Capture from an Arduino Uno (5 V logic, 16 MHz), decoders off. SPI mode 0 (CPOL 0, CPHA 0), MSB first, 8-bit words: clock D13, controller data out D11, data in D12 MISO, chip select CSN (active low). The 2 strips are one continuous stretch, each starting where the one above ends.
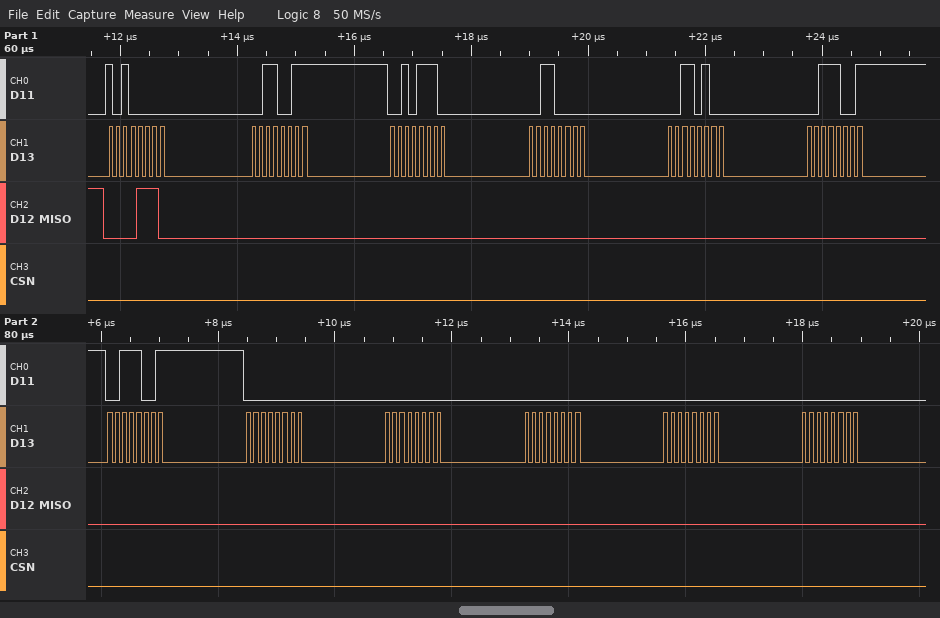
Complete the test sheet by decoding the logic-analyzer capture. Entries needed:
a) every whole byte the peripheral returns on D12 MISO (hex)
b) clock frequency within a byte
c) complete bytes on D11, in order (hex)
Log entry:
0E 00 00 00 00 00 00 00 00 00 00 00
8 MHz
A0 33 2E 30 34 39 39 00 00 00 00 00
